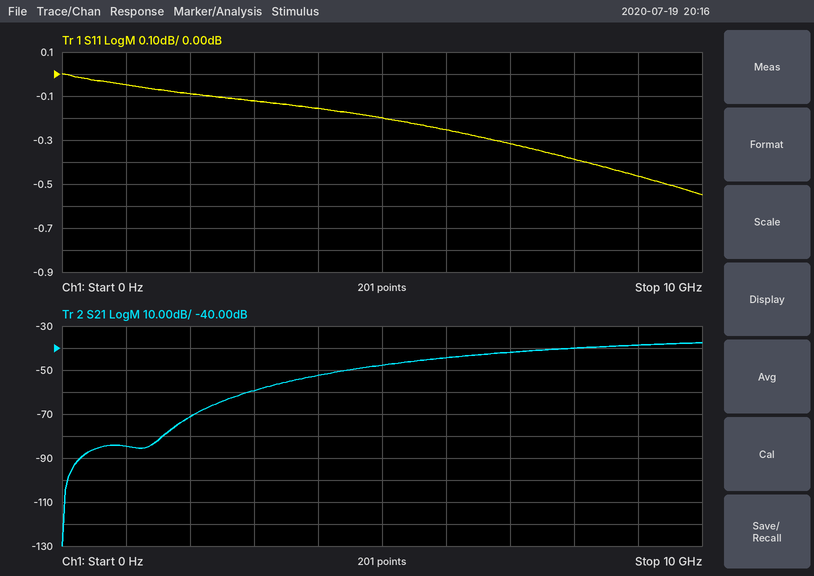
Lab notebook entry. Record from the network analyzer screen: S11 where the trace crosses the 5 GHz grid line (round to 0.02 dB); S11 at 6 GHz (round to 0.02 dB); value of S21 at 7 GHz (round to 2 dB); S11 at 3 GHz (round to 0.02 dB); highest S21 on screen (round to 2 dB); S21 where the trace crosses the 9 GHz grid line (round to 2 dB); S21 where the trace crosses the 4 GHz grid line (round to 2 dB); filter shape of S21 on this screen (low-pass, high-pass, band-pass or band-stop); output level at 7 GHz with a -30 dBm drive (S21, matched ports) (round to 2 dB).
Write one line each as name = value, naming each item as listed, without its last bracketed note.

S11 where the trace crosses the 5 GHz grid line = -0.20 dB
S11 at 6 GHz = -0.26 dB
value of S21 at 7 GHz = -42 dB
S11 at 3 GHz = -0.12 dB
highest S21 on screen = -38 dB
S21 where the trace crosses the 9 GHz grid line = -38 dB
S21 where the trace crosses the 4 GHz grid line = -52 dB
filter shape of S21 on this screen = high-pass
output level at 7 GHz with a -30 dBm drive (S21, matched ports) = -72 dBm
